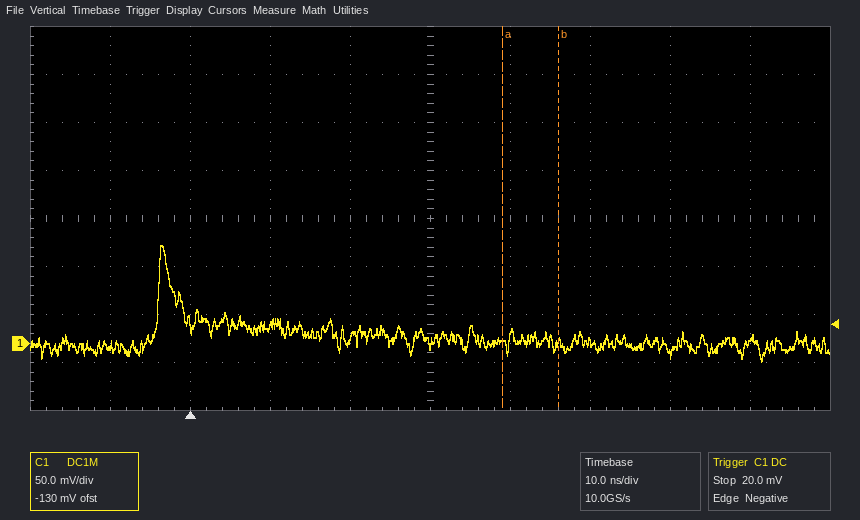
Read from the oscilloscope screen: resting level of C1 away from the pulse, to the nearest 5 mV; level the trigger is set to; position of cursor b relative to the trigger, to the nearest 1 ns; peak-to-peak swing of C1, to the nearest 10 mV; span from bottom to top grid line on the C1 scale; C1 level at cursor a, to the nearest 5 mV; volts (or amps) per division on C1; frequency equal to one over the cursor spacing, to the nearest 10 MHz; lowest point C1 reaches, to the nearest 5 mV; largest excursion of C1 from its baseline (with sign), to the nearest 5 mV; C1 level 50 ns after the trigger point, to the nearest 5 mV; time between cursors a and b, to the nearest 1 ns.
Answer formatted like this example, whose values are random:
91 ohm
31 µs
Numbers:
0 mV
20.0 mV
+46 ns
120 mV
400 mV
0 mV
50 mV
140 MHz
-20 mV
+100 mV
0 mV
7 ns
